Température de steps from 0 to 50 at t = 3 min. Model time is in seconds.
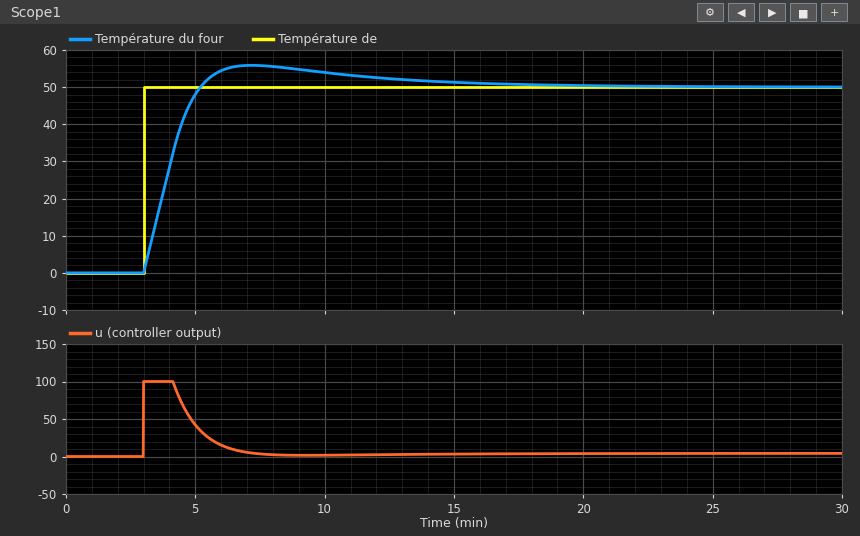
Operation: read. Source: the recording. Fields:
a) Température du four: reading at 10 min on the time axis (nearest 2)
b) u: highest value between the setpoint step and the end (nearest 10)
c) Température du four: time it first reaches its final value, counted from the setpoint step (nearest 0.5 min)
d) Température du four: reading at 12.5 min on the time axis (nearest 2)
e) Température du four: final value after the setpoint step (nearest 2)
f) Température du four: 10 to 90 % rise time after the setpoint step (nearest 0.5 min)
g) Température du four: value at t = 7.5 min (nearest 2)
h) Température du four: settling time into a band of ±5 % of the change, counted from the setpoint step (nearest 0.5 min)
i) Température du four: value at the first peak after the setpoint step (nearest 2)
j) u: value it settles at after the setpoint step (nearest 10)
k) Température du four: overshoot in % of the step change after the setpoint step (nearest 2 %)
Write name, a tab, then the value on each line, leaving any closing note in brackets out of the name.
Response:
Température du four: reading at 10 min on the time axis	54
u: highest value between the setpoint step and the end	100
Température du four: time it first reaches its final value, counted from the setpoint step	2.0 min
Température du four: reading at 12.5 min on the time axis	52
Température du four: final value after the setpoint step	50
Température du four: 10 to 90 % rise time after the setpoint step	1.5 min
Température du four: value at t = 7.5 min	56
Température du four: settling time into a band of ±5 % of the change, counted from the setpoint step	9.0 min
Température du four: value at the first peak after the setpoint step	56
u: value it settles at after the setpoint step	0
Température du four: overshoot in % of the step change after the setpoint step	12 %
